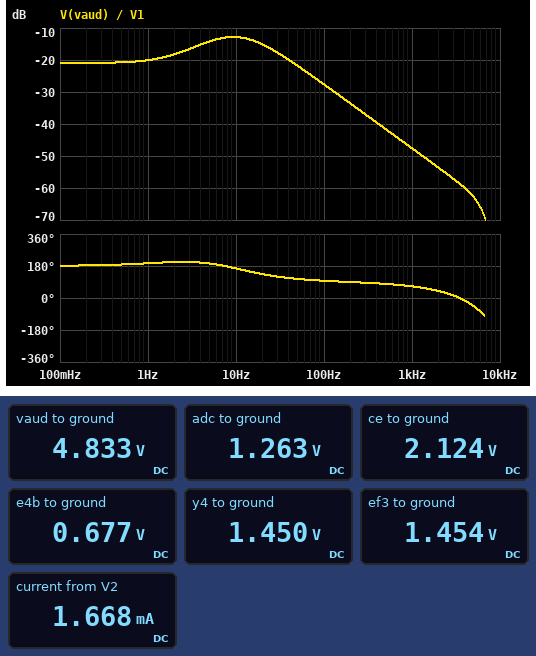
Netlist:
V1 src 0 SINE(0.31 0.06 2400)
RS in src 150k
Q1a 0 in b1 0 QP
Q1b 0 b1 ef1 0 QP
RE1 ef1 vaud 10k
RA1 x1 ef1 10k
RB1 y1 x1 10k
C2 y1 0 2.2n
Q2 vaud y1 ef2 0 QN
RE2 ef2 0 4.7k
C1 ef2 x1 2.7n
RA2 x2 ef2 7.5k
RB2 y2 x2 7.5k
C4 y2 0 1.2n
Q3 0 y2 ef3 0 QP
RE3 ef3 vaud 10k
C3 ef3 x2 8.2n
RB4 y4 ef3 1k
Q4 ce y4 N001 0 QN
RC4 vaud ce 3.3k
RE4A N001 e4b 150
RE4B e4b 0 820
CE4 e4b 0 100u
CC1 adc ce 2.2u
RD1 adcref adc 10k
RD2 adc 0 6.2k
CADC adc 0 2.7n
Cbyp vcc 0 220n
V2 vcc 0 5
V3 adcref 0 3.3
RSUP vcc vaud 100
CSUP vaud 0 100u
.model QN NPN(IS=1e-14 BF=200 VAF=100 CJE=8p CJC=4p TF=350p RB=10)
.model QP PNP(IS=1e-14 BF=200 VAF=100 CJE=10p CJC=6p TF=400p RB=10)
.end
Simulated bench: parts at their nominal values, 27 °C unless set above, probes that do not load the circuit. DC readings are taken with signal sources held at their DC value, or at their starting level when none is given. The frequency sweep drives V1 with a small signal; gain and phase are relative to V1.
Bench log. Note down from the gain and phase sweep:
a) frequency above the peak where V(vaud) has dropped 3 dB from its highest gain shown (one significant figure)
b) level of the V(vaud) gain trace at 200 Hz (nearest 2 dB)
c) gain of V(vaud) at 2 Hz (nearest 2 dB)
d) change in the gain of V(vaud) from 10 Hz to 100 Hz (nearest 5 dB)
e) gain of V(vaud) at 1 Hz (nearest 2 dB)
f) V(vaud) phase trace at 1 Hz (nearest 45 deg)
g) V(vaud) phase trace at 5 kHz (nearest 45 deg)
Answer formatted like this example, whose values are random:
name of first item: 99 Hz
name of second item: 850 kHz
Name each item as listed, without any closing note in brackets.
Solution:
frequency above the peak where V(vaud) has dropped 3 dB from its highest gain shown: 20 Hz
level of the V(vaud) gain trace at 200 Hz: -34 dB
gain of V(vaud) at 2 Hz: -18 dB
change in the gain of V(vaud) from 10 Hz to 100 Hz: -15 dB
gain of V(vaud) at 1 Hz: -20 dB
V(vaud) phase trace at 1 Hz: 180 deg
V(vaud) phase trace at 5 kHz: -45 deg
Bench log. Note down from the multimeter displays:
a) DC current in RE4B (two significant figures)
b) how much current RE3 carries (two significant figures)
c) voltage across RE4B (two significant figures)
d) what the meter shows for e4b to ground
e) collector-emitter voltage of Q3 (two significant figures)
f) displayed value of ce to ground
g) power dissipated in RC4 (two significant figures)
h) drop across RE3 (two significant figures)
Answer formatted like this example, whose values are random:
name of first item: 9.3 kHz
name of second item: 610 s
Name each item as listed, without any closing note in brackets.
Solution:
DC current in RE4B: 830 µA
how much current RE3 carries: 340 µA
voltage across RE4B: 680 mV
what the meter shows for e4b to ground: 0.677 V
collector-emitter voltage of Q3: -1.5 V
displayed value of ce to ground: 2.124 V
power dissipated in RC4: 2.2 mW
drop across RE3: 3.4 V
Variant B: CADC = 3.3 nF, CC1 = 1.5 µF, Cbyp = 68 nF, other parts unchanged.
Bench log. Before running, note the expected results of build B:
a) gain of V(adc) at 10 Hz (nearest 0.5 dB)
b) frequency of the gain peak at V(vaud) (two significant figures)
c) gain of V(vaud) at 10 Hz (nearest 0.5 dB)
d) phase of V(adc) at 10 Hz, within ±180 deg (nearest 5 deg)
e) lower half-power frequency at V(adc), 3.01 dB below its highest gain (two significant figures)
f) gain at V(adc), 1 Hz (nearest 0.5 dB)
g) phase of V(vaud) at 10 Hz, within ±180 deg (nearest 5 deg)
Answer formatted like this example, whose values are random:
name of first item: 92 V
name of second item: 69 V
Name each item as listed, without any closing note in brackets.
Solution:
gain of V(adc) at 10 Hz: 10.5 dB
frequency of the gain peak at V(vaud): 10 Hz
gain of V(vaud) at 10 Hz: -12.0 dB
phase of V(adc) at 10 Hz, within ±180 deg: -90 deg
lower half-power frequency at V(adc), 3.01 dB below its highest gain: 20 Hz
gain at V(adc), 1 Hz: -18.0 dB
phase of V(vaud) at 10 Hz, within ±180 deg: 170 deg
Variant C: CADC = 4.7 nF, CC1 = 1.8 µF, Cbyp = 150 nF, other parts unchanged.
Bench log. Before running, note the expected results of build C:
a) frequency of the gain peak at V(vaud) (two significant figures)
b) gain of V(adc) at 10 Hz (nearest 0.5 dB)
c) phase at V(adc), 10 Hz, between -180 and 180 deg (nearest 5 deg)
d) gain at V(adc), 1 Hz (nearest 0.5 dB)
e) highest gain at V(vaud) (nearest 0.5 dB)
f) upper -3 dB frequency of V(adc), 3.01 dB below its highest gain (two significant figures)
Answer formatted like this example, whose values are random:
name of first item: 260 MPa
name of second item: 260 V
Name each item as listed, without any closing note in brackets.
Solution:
frequency of the gain peak at V(vaud): 9.7 Hz
gain of V(adc) at 10 Hz: 11.5 dB
phase at V(adc), 10 Hz, between -180 and 180 deg: -95 deg
gain at V(adc), 1 Hz: -16.5 dB
highest gain at V(vaud): -12.5 dB
upper -3 dB frequency of V(adc), 3.01 dB below its highest gain: 6.0 kHz
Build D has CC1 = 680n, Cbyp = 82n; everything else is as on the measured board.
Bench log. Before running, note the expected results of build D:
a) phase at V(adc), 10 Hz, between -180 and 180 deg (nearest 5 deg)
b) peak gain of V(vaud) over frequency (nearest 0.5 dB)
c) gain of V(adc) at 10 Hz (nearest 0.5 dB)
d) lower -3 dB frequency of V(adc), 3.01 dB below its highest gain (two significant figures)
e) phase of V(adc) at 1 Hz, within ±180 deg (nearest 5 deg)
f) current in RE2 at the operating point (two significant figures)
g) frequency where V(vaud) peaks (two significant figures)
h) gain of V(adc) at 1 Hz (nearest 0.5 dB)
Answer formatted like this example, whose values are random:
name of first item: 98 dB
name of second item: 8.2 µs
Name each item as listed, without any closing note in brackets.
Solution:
phase at V(adc), 10 Hz, between -180 and 180 deg: -75 deg
peak gain of V(vaud) over frequency: -11.0 dB
gain of V(adc) at 10 Hz: 5.0 dB
lower -3 dB frequency of V(adc), 3.01 dB below its highest gain: 36 Hz
phase of V(adc) at 1 Hz, within ±180 deg: -70 deg
current in RE2 at the operating point: 170 µA
frequency where V(vaud) peaks: 12 Hz
gain of V(adc) at 1 Hz: -25.0 dB
